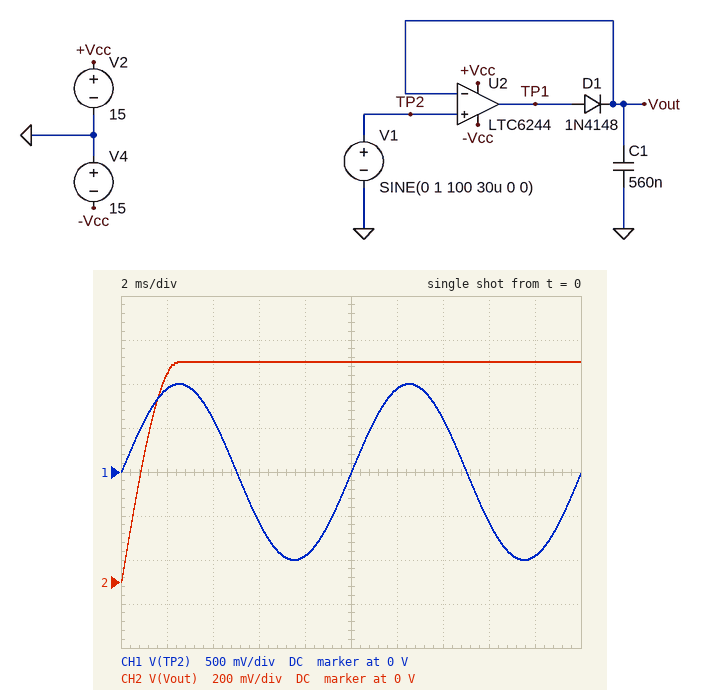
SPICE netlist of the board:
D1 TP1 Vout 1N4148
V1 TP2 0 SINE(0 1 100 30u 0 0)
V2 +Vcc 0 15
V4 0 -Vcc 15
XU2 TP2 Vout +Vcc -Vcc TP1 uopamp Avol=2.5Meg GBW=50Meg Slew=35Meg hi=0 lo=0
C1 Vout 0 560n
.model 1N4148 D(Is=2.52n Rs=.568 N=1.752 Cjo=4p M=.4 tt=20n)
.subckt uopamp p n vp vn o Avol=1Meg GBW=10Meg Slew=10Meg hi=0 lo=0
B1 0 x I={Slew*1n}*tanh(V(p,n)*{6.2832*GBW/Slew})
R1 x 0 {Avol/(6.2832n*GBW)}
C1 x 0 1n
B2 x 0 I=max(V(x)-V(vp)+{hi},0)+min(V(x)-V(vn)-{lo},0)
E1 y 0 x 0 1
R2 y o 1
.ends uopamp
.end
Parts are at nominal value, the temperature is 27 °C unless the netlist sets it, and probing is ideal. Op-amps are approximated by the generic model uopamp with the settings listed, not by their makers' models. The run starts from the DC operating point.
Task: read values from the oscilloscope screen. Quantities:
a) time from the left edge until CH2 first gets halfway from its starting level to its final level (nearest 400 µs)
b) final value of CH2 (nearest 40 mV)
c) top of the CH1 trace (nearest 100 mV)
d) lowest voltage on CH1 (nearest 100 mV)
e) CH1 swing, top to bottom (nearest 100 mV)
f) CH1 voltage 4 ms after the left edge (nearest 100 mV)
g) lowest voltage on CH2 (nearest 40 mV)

800 µs
1.00 V
1.0 V
-1.0 V
2.0 V
600 mV
0 V
